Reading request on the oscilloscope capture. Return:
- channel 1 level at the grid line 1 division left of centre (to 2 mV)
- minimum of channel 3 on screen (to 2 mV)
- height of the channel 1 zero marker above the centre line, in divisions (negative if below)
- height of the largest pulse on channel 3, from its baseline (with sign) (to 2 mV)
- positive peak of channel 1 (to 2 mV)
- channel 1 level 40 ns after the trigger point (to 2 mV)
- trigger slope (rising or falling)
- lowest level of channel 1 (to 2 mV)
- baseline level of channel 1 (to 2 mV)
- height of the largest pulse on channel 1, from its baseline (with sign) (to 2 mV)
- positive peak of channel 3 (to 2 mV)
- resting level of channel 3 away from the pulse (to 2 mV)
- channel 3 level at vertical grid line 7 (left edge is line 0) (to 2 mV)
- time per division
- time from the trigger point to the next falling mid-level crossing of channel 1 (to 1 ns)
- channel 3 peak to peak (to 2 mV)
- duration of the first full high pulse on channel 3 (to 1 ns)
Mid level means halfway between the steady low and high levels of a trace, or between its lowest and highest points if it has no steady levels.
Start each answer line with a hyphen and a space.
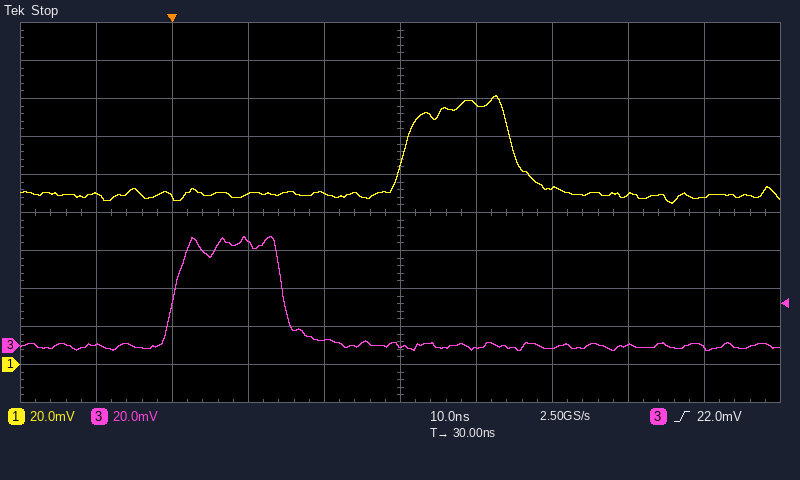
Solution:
- 90 mV
- -2 mV
- -4.0 div
- +58 mV
- 142 mV
- 138 mV
- rising
- 84 mV
- 90 mV
- +52 mV
- 58 mV
- 0 mV
- -2 mV
- 10 ns
- 45 ns
- 60 mV
- 14 ns
